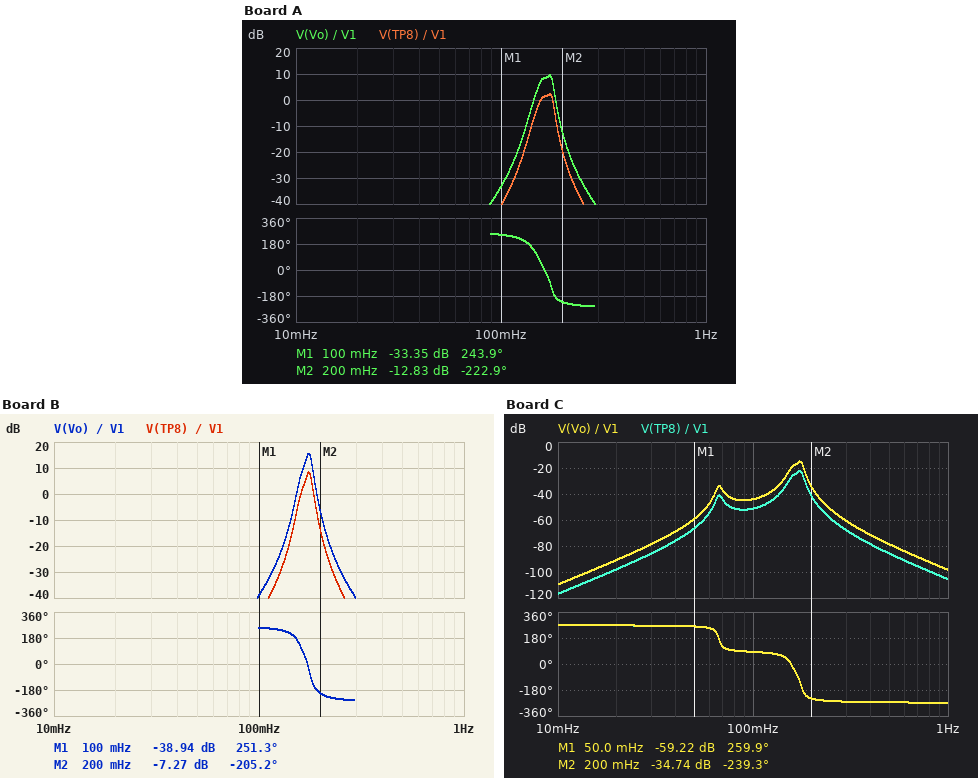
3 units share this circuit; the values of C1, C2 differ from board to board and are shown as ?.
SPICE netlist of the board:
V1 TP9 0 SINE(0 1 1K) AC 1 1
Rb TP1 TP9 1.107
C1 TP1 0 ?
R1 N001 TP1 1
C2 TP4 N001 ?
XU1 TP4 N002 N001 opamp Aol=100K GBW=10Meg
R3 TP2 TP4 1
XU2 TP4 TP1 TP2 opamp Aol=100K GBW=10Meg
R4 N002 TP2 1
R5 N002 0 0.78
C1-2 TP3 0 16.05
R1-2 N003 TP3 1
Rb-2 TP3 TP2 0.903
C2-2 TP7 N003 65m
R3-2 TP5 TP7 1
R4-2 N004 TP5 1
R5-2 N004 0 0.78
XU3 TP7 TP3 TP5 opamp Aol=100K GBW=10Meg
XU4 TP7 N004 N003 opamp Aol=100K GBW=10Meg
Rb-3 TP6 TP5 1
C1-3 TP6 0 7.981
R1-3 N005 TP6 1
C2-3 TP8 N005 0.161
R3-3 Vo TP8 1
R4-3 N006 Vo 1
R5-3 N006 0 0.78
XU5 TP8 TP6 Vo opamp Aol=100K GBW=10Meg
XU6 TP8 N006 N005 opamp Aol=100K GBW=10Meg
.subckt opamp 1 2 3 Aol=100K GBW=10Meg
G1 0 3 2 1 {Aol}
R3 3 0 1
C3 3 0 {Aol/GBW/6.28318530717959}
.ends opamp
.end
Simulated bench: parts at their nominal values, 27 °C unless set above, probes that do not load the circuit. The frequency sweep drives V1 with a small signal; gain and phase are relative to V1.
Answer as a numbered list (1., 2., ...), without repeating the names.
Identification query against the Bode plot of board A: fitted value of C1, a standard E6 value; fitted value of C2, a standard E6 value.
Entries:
1. 4.7 F
2. 330 mF
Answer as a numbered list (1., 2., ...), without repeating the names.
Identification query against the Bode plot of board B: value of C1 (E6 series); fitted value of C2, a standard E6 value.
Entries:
1. 4.7 F
2. 220 mF
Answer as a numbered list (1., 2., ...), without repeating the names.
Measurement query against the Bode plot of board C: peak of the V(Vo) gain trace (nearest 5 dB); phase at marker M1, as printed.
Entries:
1. -15 dB
2. 259.9 deg
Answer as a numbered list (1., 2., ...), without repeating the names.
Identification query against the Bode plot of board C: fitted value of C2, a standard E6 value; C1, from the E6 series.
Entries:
1. 220 mF
2. 33 F
